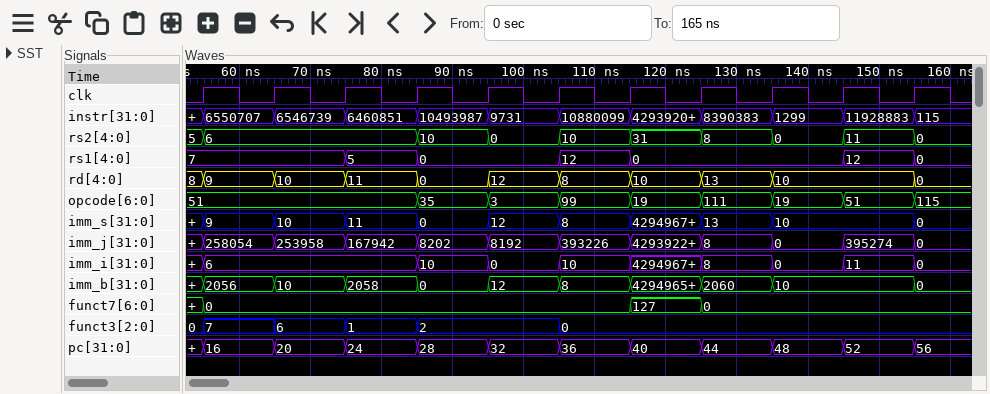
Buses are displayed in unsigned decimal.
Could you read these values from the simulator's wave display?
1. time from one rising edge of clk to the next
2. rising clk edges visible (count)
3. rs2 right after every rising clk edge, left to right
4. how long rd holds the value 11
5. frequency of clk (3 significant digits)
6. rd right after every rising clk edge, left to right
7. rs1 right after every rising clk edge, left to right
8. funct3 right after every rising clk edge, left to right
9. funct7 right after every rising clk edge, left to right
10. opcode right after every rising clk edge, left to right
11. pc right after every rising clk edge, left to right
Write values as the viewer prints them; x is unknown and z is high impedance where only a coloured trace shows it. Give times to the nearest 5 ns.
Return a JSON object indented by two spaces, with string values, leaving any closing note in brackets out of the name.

{
  "time from one rising edge of clk to the next": "10 ns",
  "rising clk edges visible": "11",
  "rs2 right after every rising clk edge, left to right": "6, 6, 6, 10, 0, 10, 31, 8, 0, 11, 0",
  "how long rd holds the value 11": "10 ns",
  "frequency of clk": "100 MHz",
  "rd right after every rising clk edge, left to right": "9, 10, 11, 0, 12, 8, 10, 13, 10, 10, 0",
  "rs1 right after every rising clk edge, left to right": "7, 7, 5, 0, 0, 12, 0, 0, 0, 12, 0",
  "funct3 right after every rising clk edge, left to right": "7, 6, 1, 2, 2, 0, 0, 0, 0, 0, 0",
  "funct7 right after every rising clk edge, left to right": "0, 0, 0, 0, 0, 0, 127, 0, 0, 0, 0",
  "opcode right after every rising clk edge, left to right": "51, 51, 51, 35, 3, 99, 19, 111, 19, 51, 115",
  "pc right after every rising clk edge, left to right": "16, 20, 24, 28, 32, 36, 40, 44, 48, 52, 56"
}
